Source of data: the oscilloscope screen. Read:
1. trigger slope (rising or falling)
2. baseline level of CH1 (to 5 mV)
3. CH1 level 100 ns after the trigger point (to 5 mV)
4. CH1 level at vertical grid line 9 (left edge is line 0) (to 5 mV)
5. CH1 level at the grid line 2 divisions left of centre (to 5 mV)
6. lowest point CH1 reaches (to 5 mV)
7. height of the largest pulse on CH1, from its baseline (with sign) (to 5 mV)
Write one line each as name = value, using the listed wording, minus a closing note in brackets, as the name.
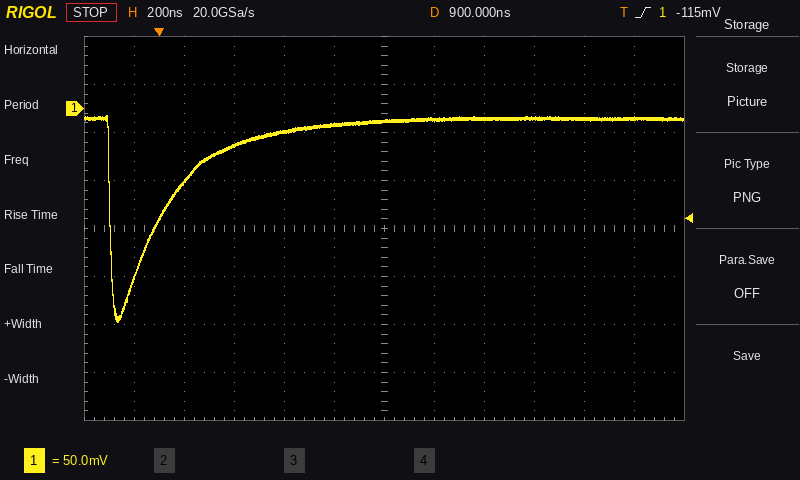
trigger slope = rising
baseline level of CH1 = -10 mV
CH1 level 100 ns after the trigger point = -75 mV
CH1 level at vertical grid line 9 (left edge is line 0) = -10 mV
CH1 level at the grid line 2 divisions left of centre = -25 mV
lowest point CH1 reaches = -220 mV
height of the largest pulse on CH1, from its baseline (with sign) = -210 mV
